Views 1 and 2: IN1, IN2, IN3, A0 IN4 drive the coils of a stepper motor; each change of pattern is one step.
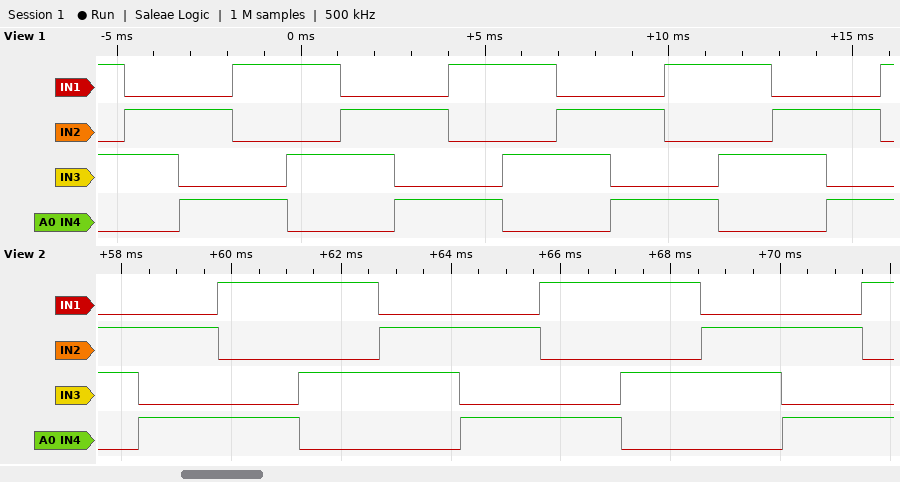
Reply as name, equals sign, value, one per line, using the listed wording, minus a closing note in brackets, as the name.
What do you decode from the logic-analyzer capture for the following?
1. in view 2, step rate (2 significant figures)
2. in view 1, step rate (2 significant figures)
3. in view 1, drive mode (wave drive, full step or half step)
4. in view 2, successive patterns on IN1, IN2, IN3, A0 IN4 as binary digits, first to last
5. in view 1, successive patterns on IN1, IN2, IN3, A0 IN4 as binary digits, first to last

in view 2, step rate = 680 steps/s
in view 1, step rate = 680 steps/s
in view 1, drive mode = full step
in view 2, successive patterns on IN1, IN2, IN3, A0 IN4 as binary digits, first to last = 0110 0101 1001 1010 0110 0101 1001 1010 0110 0101 1001
in view 1, successive patterns on IN1, IN2, IN3, A0 IN4 as binary digits, first to last = 1010 0110 0101 1001 1010 0110 0101 1001 1010 0110 0101 1001 1010 0110 0101 1001
